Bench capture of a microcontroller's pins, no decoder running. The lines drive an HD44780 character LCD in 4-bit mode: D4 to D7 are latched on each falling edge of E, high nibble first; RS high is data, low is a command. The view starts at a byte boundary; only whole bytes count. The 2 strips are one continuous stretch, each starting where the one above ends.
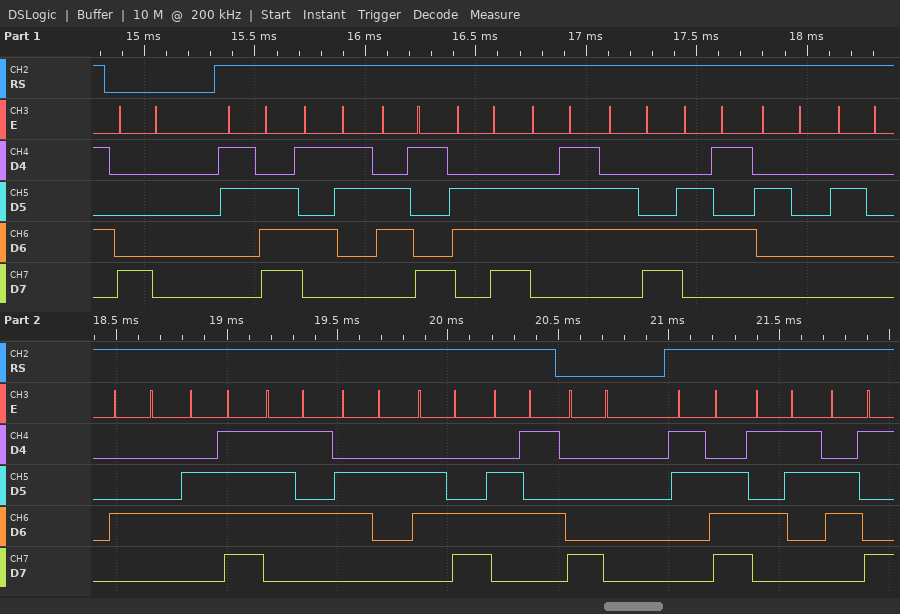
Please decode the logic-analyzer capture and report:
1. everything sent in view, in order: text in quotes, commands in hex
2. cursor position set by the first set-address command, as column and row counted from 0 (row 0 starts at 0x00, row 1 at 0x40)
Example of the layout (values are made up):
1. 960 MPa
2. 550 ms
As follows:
1. 0x80 ">Single  Double" 0x80 ">Si"
2. column 0, row 0
